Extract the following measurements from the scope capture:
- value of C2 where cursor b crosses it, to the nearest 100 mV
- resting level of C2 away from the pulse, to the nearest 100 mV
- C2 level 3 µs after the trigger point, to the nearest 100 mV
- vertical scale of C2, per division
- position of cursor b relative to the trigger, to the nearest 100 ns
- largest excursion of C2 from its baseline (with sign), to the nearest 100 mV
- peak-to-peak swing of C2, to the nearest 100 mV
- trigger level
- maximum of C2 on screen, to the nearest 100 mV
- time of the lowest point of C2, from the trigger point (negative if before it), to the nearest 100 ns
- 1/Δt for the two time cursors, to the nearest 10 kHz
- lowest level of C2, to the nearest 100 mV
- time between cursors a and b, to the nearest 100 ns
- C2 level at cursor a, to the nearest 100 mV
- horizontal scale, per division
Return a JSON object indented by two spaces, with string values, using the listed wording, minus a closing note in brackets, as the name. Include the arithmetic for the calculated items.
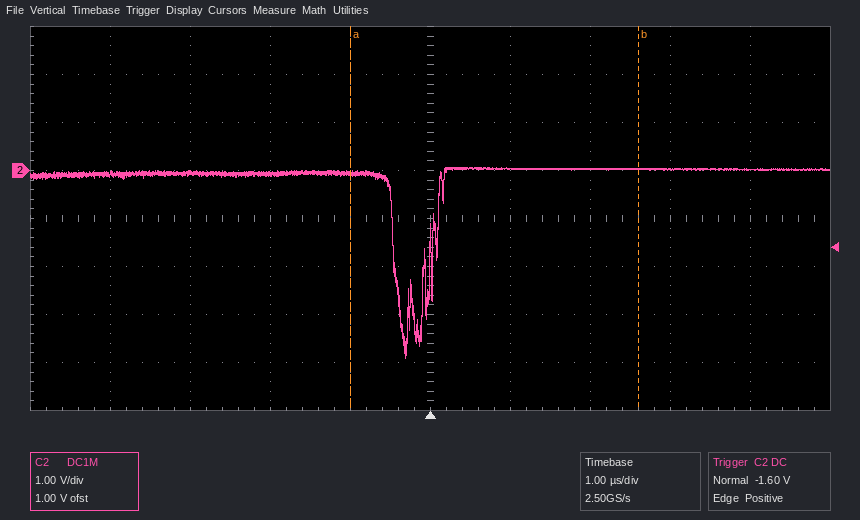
{
  "value of C2 where cursor b crosses it, to the nearest 100 mV": "0.0 V",
  "resting level of C2 away from the pulse, to the nearest 100 mV": "0.0 V",
  "C2 level 3 µs after the trigger point, to the nearest 100 mV": "0.0 V",
  "vertical scale of C2, per division": "1 V",
  "position of cursor b relative to the trigger, to the nearest 100 ns": "+2.6 µs",
  "largest excursion of C2 from its baseline (with sign), to the nearest 100 mV": "-3.9 V − (0.0 V) = -3.9 V",
  "peak-to-peak swing of C2, to the nearest 100 mV": "100 mV − (-3.9 V) = 4.0 V",
  "trigger level": "-1.60 V",
  "maximum of C2 on screen, to the nearest 100 mV": "100 mV",
  "time of the lowest point of C2, from the trigger point (negative if before it), to the nearest 100 ns": "-300 ns",
  "1/Δt for the two time cursors, to the nearest 10 kHz": "1 / 3.6 µs ≈ 280 kHz",
  "lowest level of C2, to the nearest 100 mV": "-3.9 V",
  "time between cursors a and b, to the nearest 100 ns": "3.6 µs",
  "C2 level at cursor a, to the nearest 100 mV": "-100 mV",
  "horizontal scale, per division": "1 µs"
}
